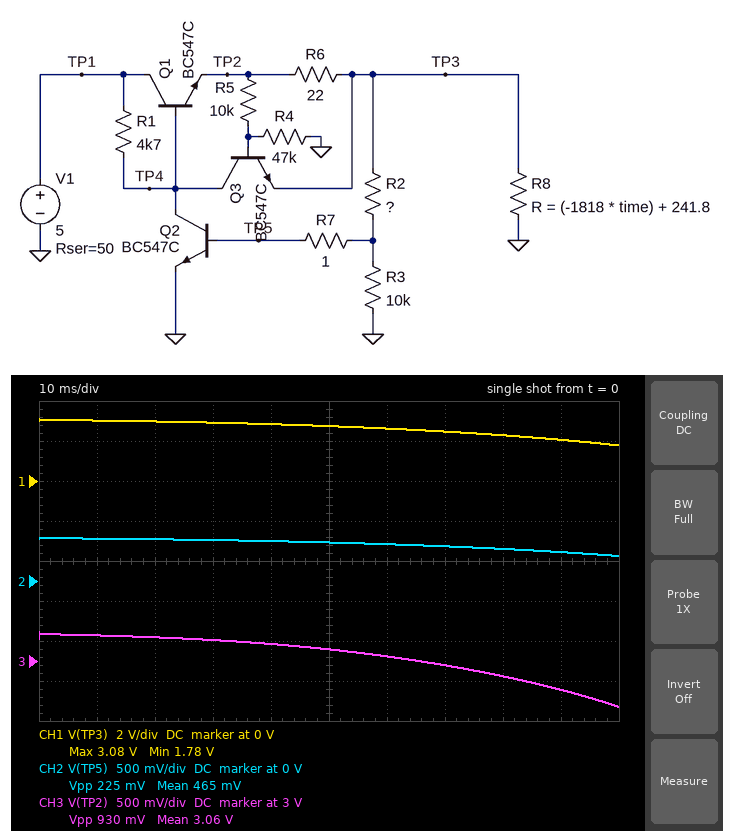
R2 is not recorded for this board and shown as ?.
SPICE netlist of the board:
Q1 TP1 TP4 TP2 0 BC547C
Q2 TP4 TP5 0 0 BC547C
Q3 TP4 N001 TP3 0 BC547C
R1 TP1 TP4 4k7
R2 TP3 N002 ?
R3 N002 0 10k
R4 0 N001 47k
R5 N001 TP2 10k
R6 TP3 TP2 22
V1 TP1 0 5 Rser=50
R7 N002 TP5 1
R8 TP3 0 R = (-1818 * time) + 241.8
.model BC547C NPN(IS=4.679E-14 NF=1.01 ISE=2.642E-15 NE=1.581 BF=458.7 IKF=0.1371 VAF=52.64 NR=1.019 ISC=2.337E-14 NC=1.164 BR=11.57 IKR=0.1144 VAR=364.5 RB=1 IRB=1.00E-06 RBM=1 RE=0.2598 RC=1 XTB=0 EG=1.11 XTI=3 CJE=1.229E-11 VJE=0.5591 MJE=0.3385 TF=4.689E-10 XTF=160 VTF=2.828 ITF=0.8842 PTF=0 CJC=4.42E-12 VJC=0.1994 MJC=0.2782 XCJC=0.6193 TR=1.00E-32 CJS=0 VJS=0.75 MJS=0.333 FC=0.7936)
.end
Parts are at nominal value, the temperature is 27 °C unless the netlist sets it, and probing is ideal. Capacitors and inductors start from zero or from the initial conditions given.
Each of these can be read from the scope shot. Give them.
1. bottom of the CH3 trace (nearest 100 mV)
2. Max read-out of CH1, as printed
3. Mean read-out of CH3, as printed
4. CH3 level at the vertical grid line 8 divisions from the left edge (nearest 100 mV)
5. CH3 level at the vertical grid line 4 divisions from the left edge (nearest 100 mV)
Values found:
2.4 V
3.08 V
3.06 V
2.8 V
3.2 V
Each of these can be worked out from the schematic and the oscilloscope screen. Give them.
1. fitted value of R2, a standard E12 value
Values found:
47 kΩ
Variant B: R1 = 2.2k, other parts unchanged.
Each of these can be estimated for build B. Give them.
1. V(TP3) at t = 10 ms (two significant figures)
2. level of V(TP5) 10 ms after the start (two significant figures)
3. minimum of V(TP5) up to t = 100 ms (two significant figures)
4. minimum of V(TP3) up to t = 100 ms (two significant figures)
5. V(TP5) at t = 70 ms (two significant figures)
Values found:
3.1 V
540 mV
330 mV
1.9 V
450 mV
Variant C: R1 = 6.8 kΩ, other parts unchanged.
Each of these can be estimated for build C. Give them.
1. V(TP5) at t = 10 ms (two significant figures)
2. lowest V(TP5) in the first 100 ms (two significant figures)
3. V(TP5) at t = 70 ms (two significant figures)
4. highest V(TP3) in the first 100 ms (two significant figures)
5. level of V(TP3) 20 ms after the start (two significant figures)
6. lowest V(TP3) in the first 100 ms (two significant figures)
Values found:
520 mV
300 mV
420 mV
3.0 V
2.9 V
1.7 V
